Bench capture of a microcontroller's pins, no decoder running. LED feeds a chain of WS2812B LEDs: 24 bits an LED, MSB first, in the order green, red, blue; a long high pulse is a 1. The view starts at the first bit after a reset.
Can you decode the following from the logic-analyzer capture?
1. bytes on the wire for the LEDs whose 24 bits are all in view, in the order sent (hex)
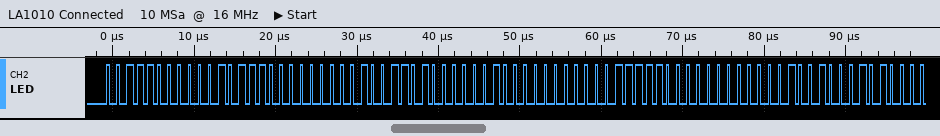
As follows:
38 17 00 4D 02 00 3E 00 12
